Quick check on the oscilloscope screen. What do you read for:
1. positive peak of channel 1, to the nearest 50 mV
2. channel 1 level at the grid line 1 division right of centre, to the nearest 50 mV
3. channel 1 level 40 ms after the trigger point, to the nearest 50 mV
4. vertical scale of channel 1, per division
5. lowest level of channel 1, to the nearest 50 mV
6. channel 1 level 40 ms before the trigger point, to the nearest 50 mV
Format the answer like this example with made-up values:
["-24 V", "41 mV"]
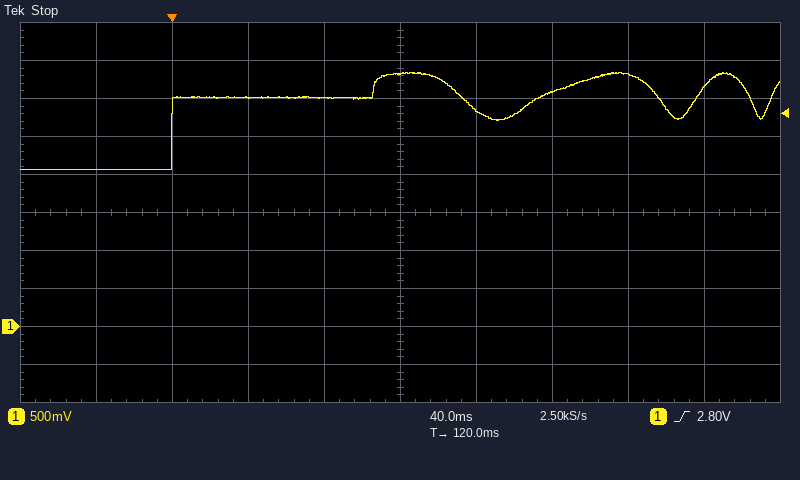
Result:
["3.35 V", "2.85 V", "3.00 V", "500 mV", "2.05 V", "2.05 V"]
